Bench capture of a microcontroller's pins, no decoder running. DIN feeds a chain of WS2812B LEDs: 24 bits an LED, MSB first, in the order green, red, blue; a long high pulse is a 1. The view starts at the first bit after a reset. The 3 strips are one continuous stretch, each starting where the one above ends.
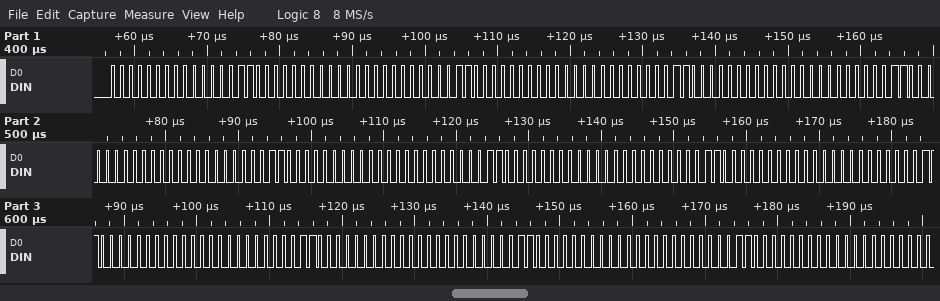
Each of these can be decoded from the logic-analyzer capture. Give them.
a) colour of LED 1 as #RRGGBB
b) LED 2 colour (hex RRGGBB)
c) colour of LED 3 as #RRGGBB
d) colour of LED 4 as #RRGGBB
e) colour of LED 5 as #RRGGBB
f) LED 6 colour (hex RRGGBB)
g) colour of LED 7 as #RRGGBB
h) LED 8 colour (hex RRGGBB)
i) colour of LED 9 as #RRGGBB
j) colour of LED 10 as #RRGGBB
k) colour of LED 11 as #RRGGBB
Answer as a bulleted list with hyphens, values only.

- #030000
- #030000
- #030000
- #030000
- #030000
- #030000
- #030000
- #030000
- #030000
- #030000
- #030000
